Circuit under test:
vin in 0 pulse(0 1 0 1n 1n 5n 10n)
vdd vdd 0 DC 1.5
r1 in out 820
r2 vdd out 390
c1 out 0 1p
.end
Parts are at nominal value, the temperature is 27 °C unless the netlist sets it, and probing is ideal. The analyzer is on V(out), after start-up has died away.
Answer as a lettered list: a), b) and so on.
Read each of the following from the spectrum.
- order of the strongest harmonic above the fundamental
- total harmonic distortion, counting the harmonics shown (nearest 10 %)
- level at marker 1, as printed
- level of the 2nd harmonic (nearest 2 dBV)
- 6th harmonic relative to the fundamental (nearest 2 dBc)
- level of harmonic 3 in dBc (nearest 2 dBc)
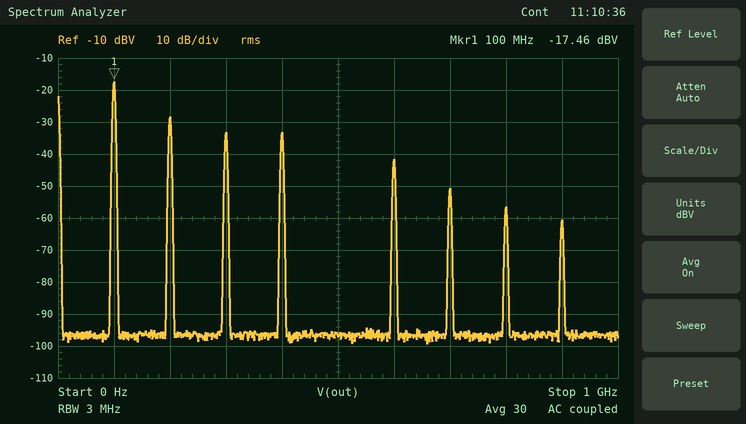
a) 2
b) 40 %
c) -17.46 dBV
d) -28 dBV
e) -24 dBc
f) -16 dBc
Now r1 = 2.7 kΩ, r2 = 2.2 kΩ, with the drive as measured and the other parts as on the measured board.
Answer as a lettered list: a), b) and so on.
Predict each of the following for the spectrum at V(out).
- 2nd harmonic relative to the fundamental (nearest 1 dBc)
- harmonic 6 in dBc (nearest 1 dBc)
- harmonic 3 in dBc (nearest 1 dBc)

a) -14 dBc
b) -33 dBc
c) -21 dBc
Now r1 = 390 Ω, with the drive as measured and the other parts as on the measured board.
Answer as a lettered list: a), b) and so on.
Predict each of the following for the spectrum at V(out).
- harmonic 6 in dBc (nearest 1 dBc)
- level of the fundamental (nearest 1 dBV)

a) -23 dBc
b) -14 dBV
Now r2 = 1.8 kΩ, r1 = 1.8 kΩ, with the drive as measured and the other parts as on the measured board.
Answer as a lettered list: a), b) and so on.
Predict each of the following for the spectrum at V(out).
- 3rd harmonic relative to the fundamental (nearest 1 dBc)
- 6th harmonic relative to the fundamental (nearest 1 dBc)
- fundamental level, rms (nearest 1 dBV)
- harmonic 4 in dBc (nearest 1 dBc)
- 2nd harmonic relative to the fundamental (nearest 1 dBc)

a) -20 dBc
b) -31 dBc
c) -15 dBV
d) -21 dBc
e) -13 dBc
